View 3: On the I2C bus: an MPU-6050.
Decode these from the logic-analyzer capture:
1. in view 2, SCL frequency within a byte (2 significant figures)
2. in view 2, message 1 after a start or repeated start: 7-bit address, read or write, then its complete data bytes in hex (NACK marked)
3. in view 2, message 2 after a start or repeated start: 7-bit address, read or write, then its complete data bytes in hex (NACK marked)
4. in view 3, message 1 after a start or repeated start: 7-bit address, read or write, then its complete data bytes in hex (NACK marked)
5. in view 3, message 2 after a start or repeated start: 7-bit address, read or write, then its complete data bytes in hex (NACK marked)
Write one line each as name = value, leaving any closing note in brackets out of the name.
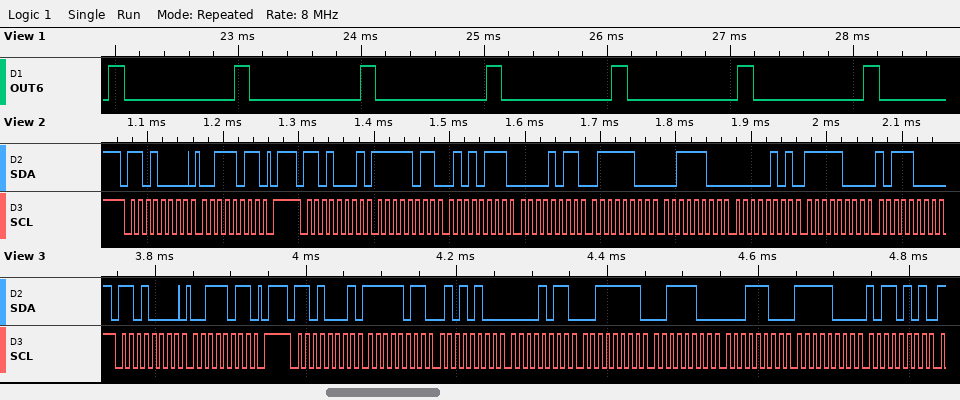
in view 2, SCL frequency within a byte = 100 kHz
in view 2, message 1 after a start or repeated start: 7-bit address, read or write, then its complete data bytes in hex = 0x68 write: 3B
in view 2, message 2 after a start or repeated start: 7-bit address, read or write, then its complete data bytes in hex = 0x68 read: FB 57 0B 7C 3C 05 F8 B8
in view 3, message 1 after a start or repeated start: 7-bit address, read or write, then its complete data bytes in hex = 0x68 write: 3B
in view 3, message 2 after a start or repeated start: 7-bit address, read or write, then its complete data bytes in hex = 0x68 read: FB 54 0B 3F 3C 1C F8 B5
